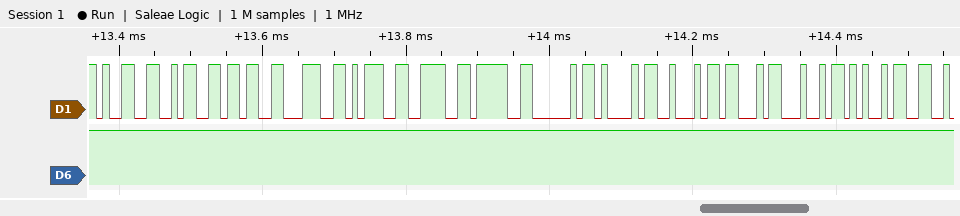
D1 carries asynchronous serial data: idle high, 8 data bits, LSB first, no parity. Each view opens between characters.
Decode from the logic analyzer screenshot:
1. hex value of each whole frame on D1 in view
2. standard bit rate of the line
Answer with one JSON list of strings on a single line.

["99, 9A, 9B, 9C, 9D, 9E, 9F, A0, A1, A2, A3, A4, A5", "115200 baud"]
